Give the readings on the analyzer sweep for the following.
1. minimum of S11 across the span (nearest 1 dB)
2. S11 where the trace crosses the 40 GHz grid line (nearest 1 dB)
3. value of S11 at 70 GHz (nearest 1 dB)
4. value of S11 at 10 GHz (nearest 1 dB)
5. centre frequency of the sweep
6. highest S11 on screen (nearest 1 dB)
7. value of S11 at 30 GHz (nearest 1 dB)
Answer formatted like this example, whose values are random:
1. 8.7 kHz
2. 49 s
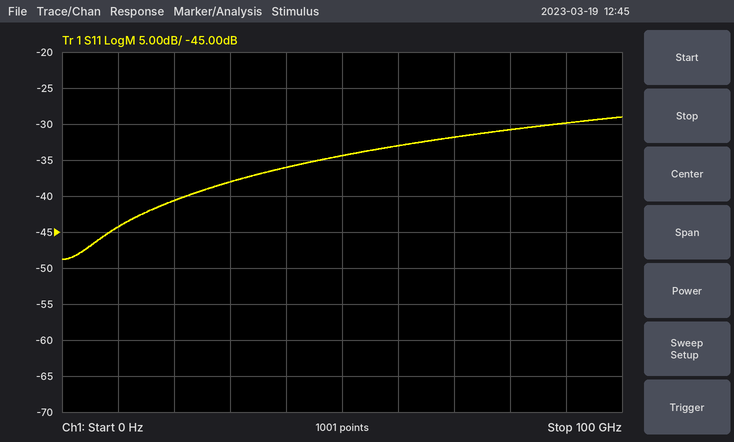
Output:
1. -49 dB
2. -36 dB
3. -32 dB
4. -44 dB
5. 50 GHz
6. -29 dB
7. -38 dB
